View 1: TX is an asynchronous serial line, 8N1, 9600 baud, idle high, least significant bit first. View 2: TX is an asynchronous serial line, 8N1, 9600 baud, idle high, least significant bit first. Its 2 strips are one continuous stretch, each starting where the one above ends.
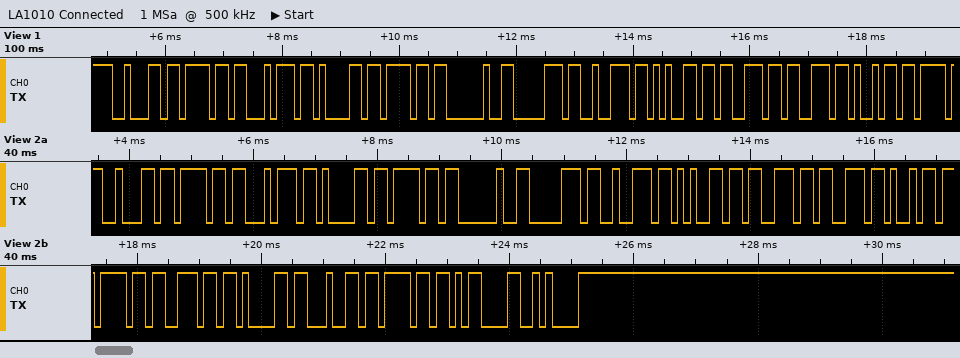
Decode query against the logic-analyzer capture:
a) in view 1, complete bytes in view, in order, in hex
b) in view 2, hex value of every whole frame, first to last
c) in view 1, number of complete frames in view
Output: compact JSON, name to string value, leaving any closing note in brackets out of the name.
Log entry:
{"in view 1, complete bytes in view, in order, in hex": "62 6F 74 61 6F 20 70 72 65 73 73 69", "in view 2, hex value of every whole frame, first to last": "62 6F 74 61 6F 20 70 72 65 73 73 69 6F 6E 61 64 6F 0D 0A", "in view 1, number of complete frames in view": "12"}
